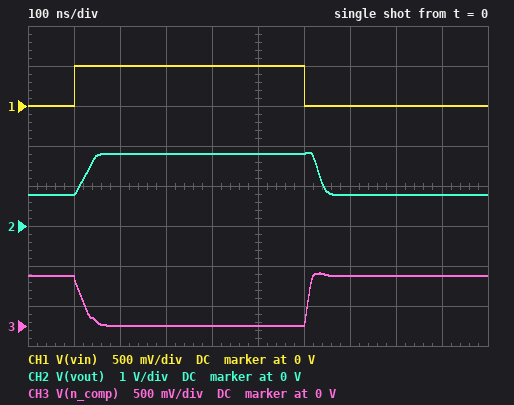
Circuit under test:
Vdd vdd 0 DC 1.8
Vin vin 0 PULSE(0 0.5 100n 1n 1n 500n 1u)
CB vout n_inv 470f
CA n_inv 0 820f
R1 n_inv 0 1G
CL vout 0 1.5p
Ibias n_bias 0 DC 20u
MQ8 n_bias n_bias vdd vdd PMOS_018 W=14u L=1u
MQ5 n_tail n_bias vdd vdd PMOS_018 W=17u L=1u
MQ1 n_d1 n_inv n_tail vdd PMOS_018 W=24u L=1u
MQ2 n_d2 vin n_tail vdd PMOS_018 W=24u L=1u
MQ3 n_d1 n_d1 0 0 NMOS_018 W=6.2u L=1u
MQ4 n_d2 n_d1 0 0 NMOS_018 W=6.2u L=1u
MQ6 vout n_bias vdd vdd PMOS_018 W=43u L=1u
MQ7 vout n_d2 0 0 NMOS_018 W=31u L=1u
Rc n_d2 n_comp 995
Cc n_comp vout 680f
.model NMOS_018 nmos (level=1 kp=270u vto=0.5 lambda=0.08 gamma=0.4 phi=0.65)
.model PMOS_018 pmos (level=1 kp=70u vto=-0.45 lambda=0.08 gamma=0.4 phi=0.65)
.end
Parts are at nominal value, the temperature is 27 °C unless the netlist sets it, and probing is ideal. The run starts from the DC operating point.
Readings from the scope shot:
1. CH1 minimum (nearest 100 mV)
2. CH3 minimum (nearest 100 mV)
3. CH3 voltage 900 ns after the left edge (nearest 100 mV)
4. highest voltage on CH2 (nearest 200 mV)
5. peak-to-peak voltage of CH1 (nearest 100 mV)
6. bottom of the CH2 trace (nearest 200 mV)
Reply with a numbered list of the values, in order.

1. 0 V
2. 0 V
3. 600 mV
4. 1.8 V
5. 500 mV
6. 800 mV
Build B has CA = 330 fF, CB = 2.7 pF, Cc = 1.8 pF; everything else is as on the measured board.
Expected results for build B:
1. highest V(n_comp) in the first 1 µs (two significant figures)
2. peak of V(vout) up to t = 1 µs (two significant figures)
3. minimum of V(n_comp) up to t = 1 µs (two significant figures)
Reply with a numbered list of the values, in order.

1. 630 mV
2. 1.3 V
3. 580 mV
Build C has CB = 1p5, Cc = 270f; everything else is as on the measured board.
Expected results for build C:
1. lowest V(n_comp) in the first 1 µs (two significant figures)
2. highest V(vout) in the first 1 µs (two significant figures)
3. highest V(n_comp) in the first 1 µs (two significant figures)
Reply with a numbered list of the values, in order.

1. 35 mV
2. 1.7 V
3. 720 mV
